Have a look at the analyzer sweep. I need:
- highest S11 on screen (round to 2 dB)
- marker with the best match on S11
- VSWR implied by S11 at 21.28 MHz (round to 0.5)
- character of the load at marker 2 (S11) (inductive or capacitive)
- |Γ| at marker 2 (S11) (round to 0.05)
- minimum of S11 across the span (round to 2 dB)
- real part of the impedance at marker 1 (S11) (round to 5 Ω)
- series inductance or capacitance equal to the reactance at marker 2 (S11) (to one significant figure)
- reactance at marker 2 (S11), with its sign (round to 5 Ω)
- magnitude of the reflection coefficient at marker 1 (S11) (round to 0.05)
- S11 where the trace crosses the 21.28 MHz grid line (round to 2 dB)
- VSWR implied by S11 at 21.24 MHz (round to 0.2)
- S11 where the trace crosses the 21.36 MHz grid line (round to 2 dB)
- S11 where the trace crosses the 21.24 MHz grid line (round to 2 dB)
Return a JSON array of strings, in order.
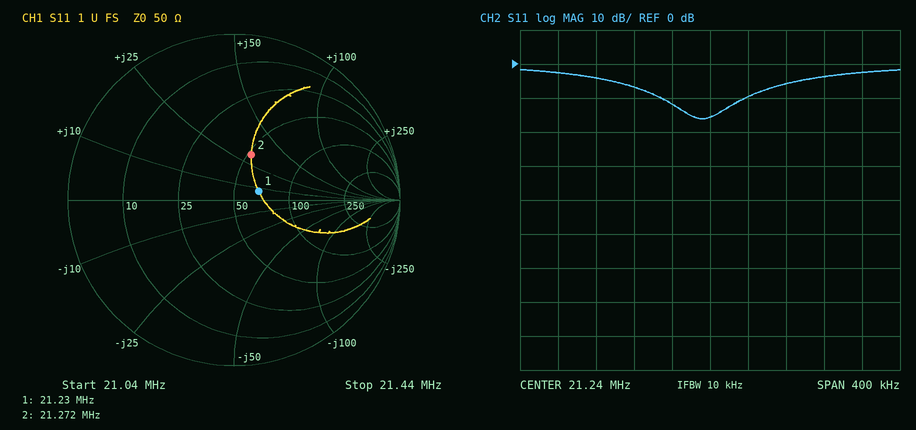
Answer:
["-2 dB", "marker 1", "2.0", "inductive", "0.30", "-16 dB", "65 Ω", "200 nH", "+30 Ω", "0.15", "-10 dB", "1.4", "-4 dB", "-16 dB"]
